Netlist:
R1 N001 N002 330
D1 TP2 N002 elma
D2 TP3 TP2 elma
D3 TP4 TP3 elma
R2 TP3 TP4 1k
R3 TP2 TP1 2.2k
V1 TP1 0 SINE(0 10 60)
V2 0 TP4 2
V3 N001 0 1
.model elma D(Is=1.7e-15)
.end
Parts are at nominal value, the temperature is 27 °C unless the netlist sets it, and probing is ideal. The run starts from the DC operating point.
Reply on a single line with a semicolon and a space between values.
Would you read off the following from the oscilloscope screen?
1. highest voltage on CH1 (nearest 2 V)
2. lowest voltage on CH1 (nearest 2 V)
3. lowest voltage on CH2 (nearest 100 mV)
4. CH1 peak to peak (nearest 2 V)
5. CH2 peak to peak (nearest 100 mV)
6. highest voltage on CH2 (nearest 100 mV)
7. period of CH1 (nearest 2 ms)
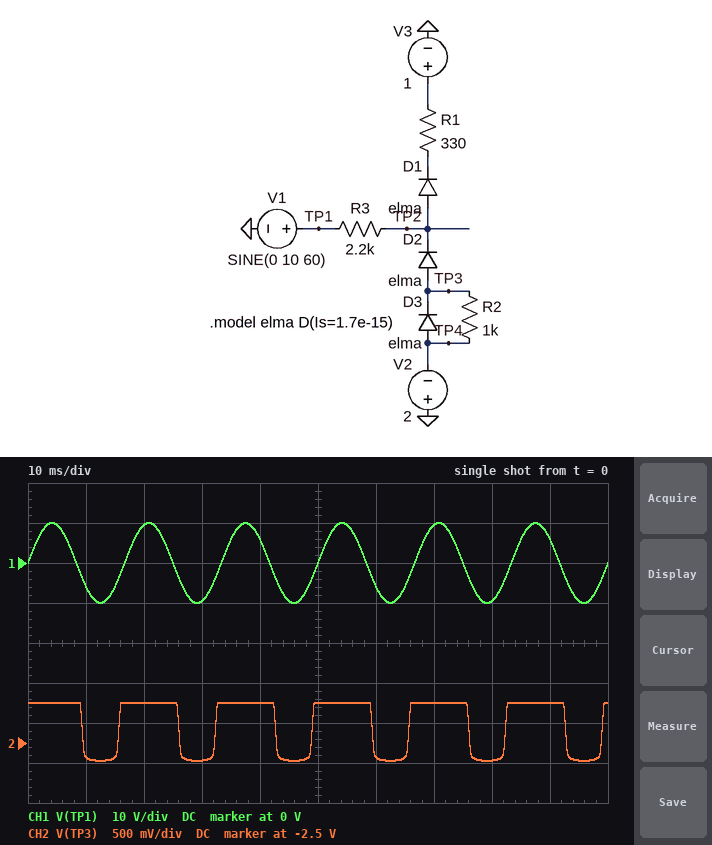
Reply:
10 V; -10 V; -2.7 V; 20 V; 700 mV; -2.0 V; 16 ms
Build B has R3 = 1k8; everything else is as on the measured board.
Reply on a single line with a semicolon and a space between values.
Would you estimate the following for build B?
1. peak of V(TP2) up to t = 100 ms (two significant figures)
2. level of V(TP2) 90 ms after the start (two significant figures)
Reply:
3.0 V; 2.4 V
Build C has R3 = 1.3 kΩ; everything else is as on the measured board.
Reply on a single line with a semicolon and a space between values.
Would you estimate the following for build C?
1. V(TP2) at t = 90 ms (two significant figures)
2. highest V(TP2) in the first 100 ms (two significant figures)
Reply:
2.6 V; 3.4 V
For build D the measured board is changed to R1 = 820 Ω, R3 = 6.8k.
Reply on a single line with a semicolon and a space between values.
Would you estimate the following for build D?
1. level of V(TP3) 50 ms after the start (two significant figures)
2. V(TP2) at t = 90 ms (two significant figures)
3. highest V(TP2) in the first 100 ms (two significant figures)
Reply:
-2.0 V; 2.1 V; 2.6 V
